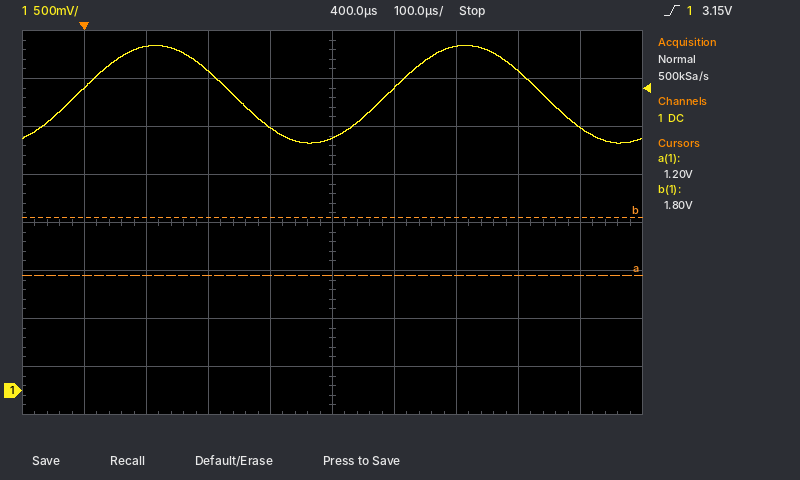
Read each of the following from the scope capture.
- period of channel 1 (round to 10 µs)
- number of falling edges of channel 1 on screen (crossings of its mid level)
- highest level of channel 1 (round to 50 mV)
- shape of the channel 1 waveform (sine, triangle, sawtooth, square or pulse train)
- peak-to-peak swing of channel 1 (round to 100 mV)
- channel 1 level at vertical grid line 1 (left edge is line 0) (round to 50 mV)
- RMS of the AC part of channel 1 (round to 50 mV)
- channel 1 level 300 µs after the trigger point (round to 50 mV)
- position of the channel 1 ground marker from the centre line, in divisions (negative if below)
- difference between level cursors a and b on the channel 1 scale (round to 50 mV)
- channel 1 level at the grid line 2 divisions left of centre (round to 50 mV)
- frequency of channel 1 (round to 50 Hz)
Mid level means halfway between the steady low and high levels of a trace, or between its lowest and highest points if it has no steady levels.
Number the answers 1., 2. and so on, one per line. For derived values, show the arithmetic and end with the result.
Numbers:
1. 500 µs
2. 2
3. 3.60 V
4. sine
5. 1.00 V
6. 3.15 V
7. 1.00 V / (2√2) ≈ 354 mV, so 350 mV to the nearest 50 mV
8. 2.75 V
9. -3.5 div
10. 600 mV
11. 3.35 V
12. 1 / 500 µs ≈ 2.00 kHz
